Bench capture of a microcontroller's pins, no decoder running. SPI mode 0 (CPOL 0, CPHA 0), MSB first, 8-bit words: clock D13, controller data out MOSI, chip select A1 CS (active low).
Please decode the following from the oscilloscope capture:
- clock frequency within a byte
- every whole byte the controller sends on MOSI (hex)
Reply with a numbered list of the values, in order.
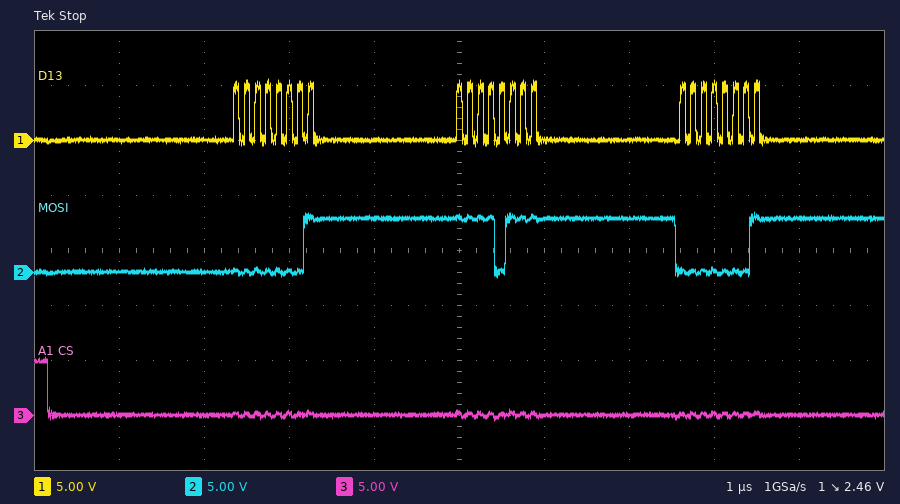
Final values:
1. 8 MHz
2. 01 F7 01
